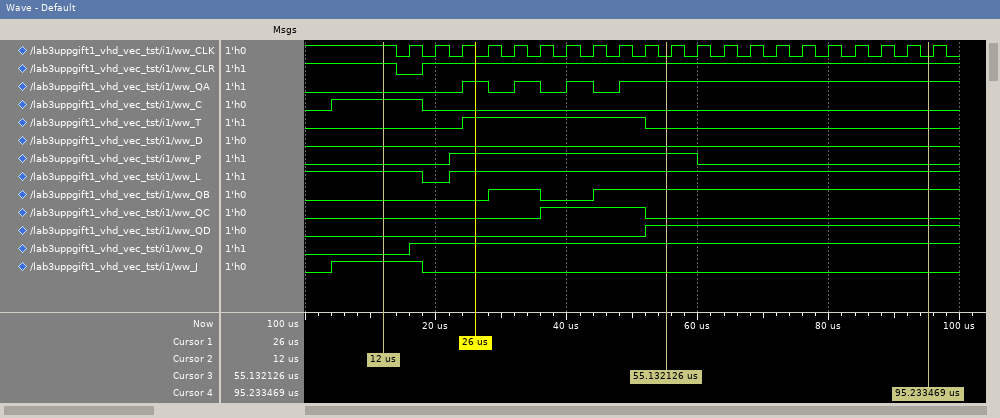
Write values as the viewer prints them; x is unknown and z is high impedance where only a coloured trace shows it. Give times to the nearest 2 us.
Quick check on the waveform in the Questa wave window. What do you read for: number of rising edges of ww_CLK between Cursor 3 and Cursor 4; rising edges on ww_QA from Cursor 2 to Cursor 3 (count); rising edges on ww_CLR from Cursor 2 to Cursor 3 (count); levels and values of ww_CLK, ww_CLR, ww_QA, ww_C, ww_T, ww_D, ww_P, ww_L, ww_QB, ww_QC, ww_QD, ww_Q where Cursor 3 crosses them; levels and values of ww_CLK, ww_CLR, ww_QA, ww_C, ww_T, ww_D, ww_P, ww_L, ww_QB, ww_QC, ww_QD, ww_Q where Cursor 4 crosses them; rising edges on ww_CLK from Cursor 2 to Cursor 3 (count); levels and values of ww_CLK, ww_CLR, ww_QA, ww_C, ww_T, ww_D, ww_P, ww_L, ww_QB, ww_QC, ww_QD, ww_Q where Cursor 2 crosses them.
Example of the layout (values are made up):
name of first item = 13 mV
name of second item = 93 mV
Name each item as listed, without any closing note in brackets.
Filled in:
number of rising edges of ww_CLK between Cursor 3 and Cursor 4 = 10
rising edges on ww_QA from Cursor 2 to Cursor 3 = 4
rising edges on ww_CLR from Cursor 2 to Cursor 3 = 1
levels and values of ww_CLK, ww_CLR, ww_QA, ww_C, ww_T, ww_D, ww_P, ww_L, ww_QB, ww_QC, ww_QD, ww_Q where Cursor 3 crosses them = ww_CLK=0, ww_CLR=1, ww_QA=1, ww_C=0, ww_T=0, ww_D=0, ww_P=1, ww_L=1, ww_QB=1, ww_QC=0, ww_QD=1, ww_Q=1
levels and values of ww_CLK, ww_CLR, ww_QA, ww_C, ww_T, ww_D, ww_P, ww_L, ww_QB, ww_QC, ww_QD, ww_Q where Cursor 4 crosses them = ww_CLK=0, ww_CLR=1, ww_QA=1, ww_C=0, ww_T=0, ww_D=0, ww_P=0, ww_L=1, ww_QB=1, ww_QC=0, ww_QD=1, ww_Q=1
rising edges on ww_CLK from Cursor 2 to Cursor 3 = 10
levels and values of ww_CLK, ww_CLR, ww_QA, ww_C, ww_T, ww_D, ww_P, ww_L, ww_QB, ww_QC, ww_QD, ww_Q where Cursor 2 crosses them = ww_CLK=1, ww_CLR=1, ww_QA=0, ww_C=1, ww_T=0, ww_D=0, ww_P=0, ww_L=1, ww_QB=0, ww_QC=0, ww_QD=0, ww_Q=0
